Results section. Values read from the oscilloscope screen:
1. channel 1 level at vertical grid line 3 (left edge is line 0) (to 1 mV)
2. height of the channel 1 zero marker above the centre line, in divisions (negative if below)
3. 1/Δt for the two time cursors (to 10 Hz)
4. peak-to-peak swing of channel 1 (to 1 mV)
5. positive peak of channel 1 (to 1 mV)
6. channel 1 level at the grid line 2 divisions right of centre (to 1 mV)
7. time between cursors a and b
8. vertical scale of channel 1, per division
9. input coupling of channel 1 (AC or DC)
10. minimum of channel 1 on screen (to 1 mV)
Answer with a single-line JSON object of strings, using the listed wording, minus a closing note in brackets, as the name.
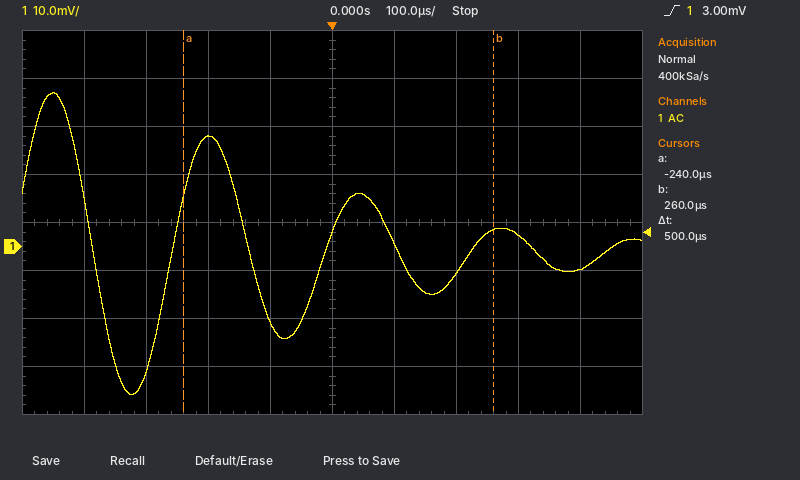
{"channel 1 level at vertical grid line 3 (left edge is line 0)": "23 mV", "height of the channel 1 zero marker above the centre line, in divisions": "-0.5 div", "1/Δt for the two time cursors": "2.00 kHz", "peak-to-peak swing of channel 1": "63 mV", "positive peak of channel 1": "32 mV", "channel 1 level at the grid line 2 divisions right of centre": "-6 mV", "time between cursors a and b": "500 µs", "vertical scale of channel 1, per division": "10 mV", "input coupling of channel 1": "AC", "minimum of channel 1 on screen": "-31 mV"}
